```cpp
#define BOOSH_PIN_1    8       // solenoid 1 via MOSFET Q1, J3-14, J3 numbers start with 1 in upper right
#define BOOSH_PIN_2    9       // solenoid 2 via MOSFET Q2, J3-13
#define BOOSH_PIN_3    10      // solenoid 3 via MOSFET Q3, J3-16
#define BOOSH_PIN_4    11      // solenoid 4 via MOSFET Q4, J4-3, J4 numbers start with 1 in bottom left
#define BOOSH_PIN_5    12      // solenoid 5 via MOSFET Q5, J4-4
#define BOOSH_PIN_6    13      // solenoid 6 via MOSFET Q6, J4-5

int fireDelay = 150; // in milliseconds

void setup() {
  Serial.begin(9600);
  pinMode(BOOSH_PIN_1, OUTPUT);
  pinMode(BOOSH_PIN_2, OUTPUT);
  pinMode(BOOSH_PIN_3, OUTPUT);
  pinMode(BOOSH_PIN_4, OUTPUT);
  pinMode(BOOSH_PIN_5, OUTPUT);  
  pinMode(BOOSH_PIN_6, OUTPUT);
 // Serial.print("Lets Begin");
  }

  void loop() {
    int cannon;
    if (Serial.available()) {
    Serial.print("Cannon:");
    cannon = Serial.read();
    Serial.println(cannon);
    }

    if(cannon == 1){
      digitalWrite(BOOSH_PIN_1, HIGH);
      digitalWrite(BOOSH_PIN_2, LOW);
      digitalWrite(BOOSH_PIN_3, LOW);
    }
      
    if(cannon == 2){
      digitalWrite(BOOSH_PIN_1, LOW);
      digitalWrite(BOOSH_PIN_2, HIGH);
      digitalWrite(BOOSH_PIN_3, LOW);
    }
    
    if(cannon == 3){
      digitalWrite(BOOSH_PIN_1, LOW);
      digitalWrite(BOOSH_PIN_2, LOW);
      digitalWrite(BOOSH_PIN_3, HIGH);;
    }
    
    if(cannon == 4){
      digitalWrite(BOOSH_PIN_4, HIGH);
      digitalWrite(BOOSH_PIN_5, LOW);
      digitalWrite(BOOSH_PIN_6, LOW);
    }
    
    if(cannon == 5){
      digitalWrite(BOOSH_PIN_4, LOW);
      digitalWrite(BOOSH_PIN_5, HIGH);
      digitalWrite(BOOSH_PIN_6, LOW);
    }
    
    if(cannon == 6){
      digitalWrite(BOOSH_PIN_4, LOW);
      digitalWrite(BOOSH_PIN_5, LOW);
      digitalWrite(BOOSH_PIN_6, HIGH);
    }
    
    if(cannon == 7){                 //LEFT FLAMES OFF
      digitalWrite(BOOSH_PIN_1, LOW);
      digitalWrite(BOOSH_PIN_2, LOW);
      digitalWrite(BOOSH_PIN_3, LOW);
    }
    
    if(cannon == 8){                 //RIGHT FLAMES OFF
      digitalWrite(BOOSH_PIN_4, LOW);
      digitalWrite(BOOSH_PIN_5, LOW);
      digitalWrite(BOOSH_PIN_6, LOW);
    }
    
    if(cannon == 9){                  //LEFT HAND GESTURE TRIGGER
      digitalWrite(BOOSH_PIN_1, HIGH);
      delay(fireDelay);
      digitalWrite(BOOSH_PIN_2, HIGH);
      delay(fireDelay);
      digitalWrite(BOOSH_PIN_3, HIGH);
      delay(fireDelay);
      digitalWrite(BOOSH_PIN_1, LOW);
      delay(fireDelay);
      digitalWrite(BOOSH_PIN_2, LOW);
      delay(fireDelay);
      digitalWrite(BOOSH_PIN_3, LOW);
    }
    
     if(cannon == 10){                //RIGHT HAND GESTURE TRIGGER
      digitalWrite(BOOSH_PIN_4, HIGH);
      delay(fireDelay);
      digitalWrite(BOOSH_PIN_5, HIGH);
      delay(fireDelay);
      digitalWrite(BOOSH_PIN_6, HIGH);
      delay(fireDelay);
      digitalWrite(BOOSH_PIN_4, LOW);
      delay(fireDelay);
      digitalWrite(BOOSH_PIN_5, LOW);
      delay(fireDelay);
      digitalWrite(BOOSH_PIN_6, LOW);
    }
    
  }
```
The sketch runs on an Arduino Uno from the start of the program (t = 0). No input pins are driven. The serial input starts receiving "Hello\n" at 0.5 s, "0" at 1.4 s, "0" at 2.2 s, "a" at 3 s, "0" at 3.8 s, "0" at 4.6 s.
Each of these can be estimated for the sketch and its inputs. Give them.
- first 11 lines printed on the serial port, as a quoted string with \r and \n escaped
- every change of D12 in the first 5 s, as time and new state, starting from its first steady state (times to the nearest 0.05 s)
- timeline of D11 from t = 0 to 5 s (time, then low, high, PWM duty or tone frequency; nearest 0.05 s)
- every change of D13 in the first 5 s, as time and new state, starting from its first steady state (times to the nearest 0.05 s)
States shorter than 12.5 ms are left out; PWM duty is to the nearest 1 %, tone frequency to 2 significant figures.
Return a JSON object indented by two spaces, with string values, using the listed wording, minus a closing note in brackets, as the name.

{
  "first 11 lines printed on the serial port, as a quoted string with \\r and \\n escaped": "\"Cannon:72\\r\\nCannon:101\\r\\nCannon:108\\r\\nCannon:108\\r\\nCannon:111\\r\\nCannon:10\\r\\nCannon:48\\r\\nCannon:48\\r\\nCannon:97\\r\\nCannon:48\\r\\nCannon:48\\r\\n\"",
  "every change of D12 in the first 5 s, as time and new state, starting from its first steady state": "0 s low; 0.65 s high; 1.1 s low",
  "timeline of D11 from t = 0 to 5 s": "0 s low; 0.5 s high; 0.95 s low",
  "every change of D13 in the first 5 s, as time and new state, starting from its first steady state": "0 s low; 0.8 s high; 1.25 s low"
}
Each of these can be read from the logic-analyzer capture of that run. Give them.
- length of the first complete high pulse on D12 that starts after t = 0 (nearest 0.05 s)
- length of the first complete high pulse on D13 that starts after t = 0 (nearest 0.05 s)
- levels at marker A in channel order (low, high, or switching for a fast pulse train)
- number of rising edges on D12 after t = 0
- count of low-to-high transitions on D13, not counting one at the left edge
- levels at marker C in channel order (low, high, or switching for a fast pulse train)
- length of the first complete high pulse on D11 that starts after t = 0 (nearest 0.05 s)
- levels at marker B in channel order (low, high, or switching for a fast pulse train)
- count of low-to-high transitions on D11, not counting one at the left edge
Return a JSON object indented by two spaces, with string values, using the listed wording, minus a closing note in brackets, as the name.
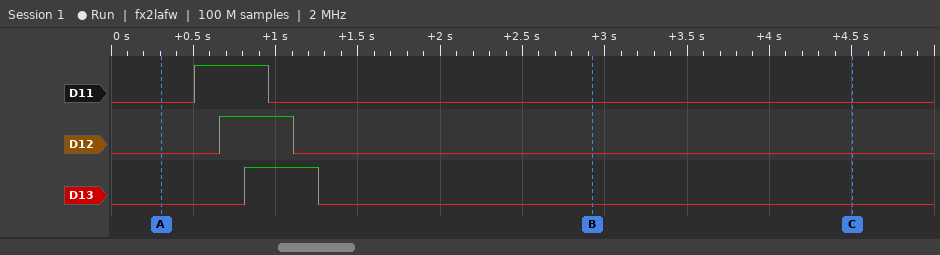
{
  "length of the first complete high pulse on D12 that starts after t = 0": "0.45 s",
  "length of the first complete high pulse on D13 that starts after t = 0": "0.45 s",
  "levels at marker A in channel order": "D11 low, D12 low, D13 low",
  "number of rising edges on D12 after t = 0": "1",
  "count of low-to-high transitions on D13, not counting one at the left edge": "1",
  "levels at marker C in channel order": "D11 low, D12 low, D13 low",
  "length of the first complete high pulse on D11 that starts after t = 0": "0.45 s",
  "levels at marker B in channel order": "D11 low, D12 low, D13 low",
  "count of low-to-high transitions on D11, not counting one at the left edge": "1"
}
